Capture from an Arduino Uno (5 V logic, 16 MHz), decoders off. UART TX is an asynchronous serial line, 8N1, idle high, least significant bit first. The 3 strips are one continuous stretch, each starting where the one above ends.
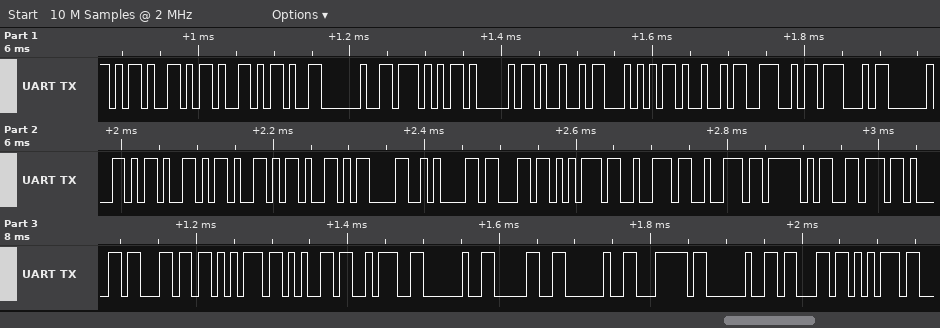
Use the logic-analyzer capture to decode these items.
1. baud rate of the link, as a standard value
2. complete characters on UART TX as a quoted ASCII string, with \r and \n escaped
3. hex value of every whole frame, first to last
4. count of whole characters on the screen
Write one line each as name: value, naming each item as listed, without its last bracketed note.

baud rate of the link, as a standard value: 115200 baud
complete characters on UART TX as a quoted ASCII string, with \r and \n escaped: "--- WAITING ---\r\ncurr_value: 0 | cu"
hex value of every whole frame, first to last: 2D 2D 2D 20 57 41 49 54 49 4E 47 20 2D 2D 2D 0D 0A 63 75 72 72 5F 76 61 6C 75 65 3A 20 30 20 7C 20 63 75
count of whole characters on the screen: 35
